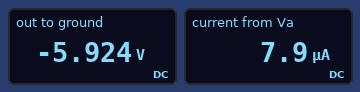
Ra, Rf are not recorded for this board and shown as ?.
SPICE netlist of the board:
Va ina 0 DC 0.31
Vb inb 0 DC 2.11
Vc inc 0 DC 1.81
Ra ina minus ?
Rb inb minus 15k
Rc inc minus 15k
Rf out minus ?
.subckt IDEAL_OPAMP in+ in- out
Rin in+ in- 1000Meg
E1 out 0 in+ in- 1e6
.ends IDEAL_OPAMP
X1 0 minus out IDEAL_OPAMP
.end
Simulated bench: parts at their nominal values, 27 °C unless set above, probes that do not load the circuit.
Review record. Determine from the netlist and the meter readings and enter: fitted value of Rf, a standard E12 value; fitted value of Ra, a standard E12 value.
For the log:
22 kΩ
39 kΩ
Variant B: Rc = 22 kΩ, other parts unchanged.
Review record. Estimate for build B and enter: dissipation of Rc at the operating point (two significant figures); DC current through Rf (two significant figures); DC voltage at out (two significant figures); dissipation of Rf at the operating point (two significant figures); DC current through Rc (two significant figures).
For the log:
150 µW
230 µA
-5.1 V
1.2 mW
82 µA
